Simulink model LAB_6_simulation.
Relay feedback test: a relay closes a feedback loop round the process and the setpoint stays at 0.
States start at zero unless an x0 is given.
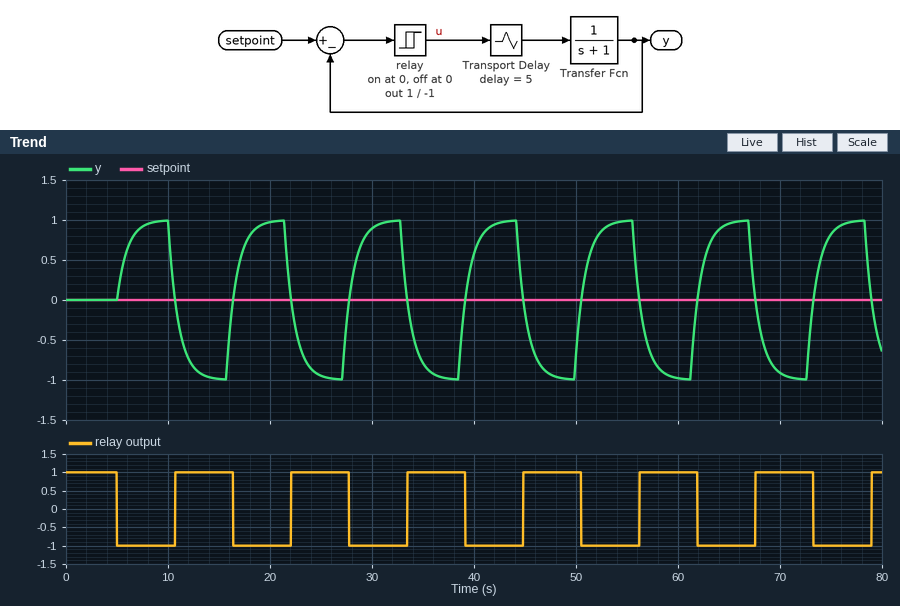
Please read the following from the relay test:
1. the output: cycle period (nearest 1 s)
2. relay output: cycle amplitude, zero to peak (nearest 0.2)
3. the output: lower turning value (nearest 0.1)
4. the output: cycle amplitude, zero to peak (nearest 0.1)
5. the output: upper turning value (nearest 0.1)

11 s
1.0
-1.0
1.0
1.0
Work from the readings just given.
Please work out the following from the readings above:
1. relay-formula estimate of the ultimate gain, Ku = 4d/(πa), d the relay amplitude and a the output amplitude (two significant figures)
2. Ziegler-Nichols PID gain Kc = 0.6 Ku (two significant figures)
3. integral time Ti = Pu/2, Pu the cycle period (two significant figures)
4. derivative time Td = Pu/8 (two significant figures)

1.3
0.78
5.5 s
1.4 s
